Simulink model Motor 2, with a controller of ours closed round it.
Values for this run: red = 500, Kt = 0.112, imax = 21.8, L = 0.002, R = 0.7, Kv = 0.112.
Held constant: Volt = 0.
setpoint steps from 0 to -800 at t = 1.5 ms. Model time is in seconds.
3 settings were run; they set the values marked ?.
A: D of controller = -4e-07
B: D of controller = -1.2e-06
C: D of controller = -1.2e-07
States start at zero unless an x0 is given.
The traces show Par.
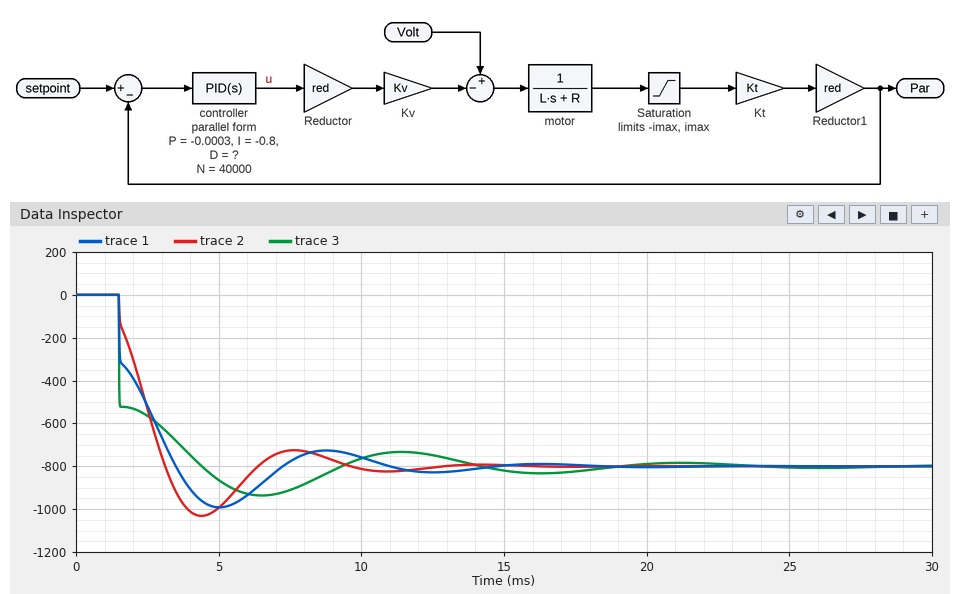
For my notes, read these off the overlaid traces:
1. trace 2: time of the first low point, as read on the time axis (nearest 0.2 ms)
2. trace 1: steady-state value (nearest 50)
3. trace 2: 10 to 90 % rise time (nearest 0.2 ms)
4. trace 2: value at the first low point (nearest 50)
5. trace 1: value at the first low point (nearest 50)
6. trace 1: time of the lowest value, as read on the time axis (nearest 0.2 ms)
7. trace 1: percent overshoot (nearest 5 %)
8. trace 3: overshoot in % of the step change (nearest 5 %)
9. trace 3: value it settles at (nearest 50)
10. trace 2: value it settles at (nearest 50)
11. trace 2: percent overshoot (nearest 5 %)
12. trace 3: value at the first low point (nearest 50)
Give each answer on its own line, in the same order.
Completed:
4.4 ms
-800
1.4 ms
-1050
-1000
5.0 ms
25 %
15 %
-800
-800
30 %
-950
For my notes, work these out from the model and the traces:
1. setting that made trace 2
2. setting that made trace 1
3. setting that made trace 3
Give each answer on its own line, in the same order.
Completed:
C
A
B
